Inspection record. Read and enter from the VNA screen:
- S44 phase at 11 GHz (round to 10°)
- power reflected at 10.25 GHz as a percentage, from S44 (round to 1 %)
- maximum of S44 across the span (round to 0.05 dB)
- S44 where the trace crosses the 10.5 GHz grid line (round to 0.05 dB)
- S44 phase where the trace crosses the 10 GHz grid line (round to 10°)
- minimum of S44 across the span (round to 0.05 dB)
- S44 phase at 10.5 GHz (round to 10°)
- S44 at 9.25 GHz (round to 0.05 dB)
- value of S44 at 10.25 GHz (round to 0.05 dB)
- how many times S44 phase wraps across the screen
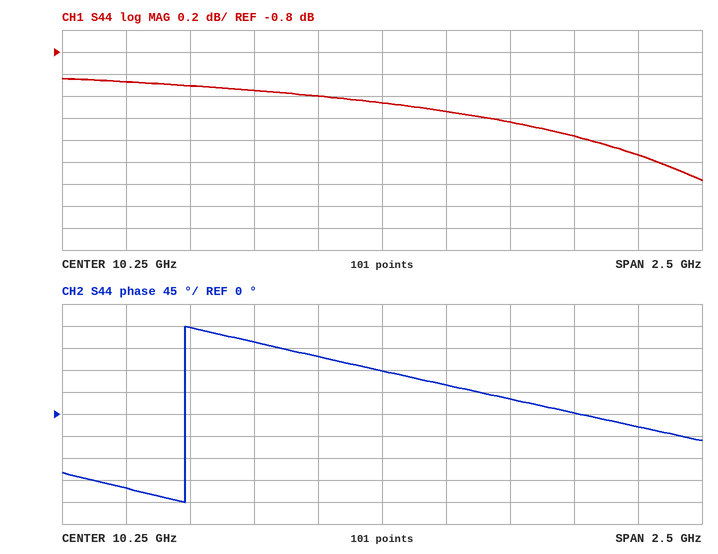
0°
75 %
-1.05 dB
-1.35 dB
120°
-1.95 dB
60°
-1.05 dB
-1.25 dB
1
